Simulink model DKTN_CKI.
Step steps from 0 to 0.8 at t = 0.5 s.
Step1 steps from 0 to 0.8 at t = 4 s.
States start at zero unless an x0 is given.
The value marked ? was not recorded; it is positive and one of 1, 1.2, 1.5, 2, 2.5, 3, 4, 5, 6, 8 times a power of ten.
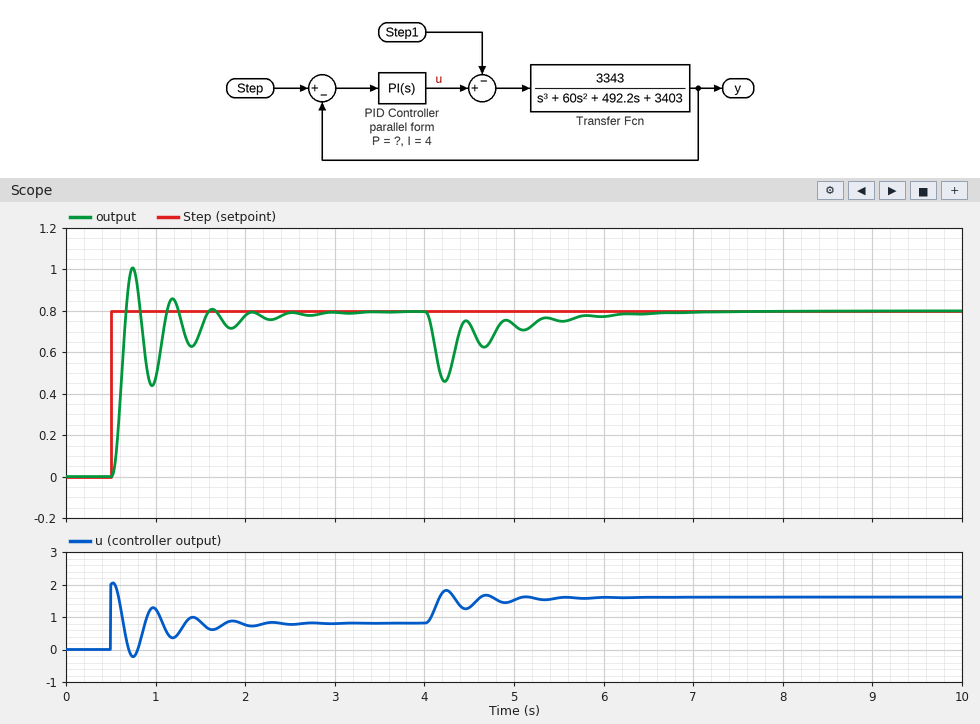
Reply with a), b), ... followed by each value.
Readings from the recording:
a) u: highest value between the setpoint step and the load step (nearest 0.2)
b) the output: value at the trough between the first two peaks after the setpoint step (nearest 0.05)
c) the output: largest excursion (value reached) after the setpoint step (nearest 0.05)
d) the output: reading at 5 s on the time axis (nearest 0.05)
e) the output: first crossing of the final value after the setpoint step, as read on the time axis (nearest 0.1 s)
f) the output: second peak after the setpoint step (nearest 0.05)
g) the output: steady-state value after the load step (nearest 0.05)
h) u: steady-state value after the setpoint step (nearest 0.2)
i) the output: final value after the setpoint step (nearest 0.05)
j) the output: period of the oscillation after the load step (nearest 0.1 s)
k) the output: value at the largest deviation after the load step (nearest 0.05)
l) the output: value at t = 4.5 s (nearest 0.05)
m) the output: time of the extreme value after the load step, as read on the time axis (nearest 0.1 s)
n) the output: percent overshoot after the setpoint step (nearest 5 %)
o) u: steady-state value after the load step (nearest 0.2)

a) 2.0
b) 0.45
c) 1.00
d) 0.75
e) 0.7 s
f) 0.85
g) 0.80
h) 0.8
i) 0.80
j) 0.4 s
k) 0.45
l) 0.75
m) 4.2 s
n) 25 %
o) 1.6
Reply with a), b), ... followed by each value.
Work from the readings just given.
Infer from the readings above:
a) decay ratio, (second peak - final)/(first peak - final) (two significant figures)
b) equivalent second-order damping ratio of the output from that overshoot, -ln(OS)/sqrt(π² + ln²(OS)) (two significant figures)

a) 0.25
b) 0.40
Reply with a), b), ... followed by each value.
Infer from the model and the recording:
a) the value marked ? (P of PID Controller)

a) 2.5
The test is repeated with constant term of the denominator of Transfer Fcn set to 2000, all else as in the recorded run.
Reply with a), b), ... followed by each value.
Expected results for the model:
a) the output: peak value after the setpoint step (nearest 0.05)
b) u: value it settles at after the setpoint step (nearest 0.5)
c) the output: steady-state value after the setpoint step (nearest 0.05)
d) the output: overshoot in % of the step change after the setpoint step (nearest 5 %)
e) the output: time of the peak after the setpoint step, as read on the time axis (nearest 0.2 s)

a) 1.10
b) 0.5
c) 0.80
d) 40 %
e) 0.8 s
